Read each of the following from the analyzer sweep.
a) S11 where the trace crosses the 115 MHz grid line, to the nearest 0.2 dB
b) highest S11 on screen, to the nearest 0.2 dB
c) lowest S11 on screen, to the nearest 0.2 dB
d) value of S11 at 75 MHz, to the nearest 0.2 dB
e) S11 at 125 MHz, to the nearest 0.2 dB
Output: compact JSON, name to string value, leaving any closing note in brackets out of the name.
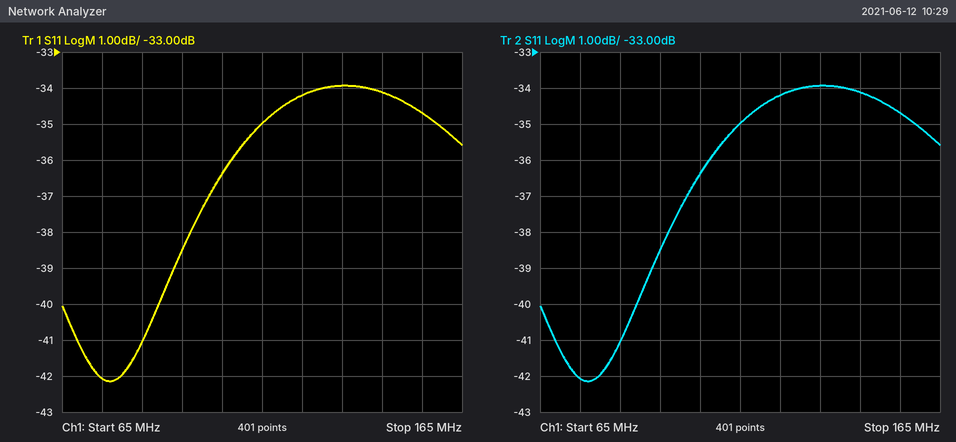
{"S11 where the trace crosses the 115 MHz grid line, to the nearest 0.2 dB": "-35.0 dB", "highest S11 on screen, to the nearest 0.2 dB": "-34.0 dB", "lowest S11 on screen, to the nearest 0.2 dB": "-42.2 dB", "value of S11 at 75 MHz, to the nearest 0.2 dB": "-42.0 dB", "S11 at 125 MHz, to the nearest 0.2 dB": "-34.2 dB"}
